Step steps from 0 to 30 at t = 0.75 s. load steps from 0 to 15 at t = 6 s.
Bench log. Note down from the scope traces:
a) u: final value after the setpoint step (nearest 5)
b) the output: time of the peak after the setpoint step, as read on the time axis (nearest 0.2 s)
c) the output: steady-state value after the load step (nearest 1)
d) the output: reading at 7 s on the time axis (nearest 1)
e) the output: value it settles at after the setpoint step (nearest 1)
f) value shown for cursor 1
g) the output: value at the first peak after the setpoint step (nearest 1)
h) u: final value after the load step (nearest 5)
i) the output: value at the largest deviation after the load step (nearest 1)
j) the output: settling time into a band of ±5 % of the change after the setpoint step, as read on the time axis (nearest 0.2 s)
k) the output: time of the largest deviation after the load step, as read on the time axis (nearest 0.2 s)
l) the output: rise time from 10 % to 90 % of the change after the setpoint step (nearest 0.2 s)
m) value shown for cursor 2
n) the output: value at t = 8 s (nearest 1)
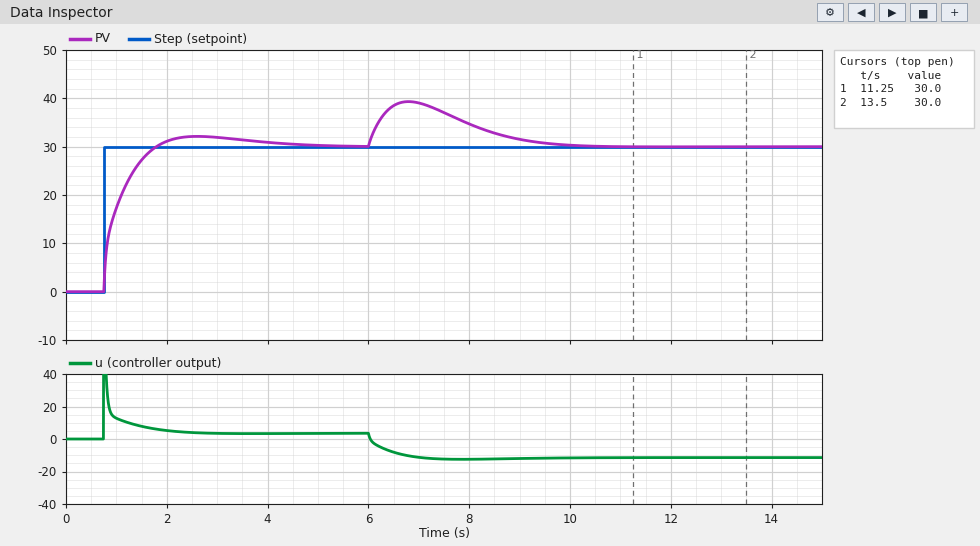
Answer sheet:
5
2.6 s
30
39
30
30.0
32
-10
39
3.4 s
6.8 s
0.8 s
30.0
35
